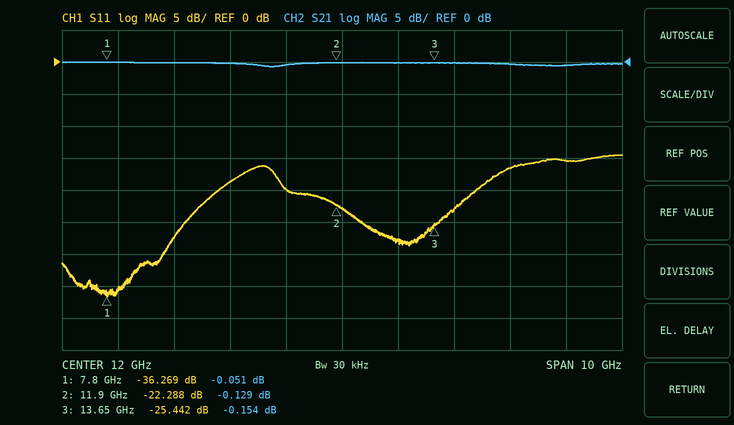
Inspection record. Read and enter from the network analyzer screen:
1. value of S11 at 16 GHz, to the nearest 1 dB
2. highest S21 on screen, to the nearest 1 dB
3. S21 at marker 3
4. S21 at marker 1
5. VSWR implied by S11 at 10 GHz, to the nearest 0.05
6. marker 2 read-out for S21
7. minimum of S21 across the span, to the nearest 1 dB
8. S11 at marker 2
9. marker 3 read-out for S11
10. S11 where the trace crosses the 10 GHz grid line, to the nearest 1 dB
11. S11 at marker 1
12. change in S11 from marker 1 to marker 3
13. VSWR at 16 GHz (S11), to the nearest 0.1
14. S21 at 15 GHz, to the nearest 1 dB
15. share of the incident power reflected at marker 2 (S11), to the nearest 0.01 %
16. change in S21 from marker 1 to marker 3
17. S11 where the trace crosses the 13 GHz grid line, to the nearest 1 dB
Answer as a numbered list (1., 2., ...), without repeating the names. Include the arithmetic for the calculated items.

1. -15 dB
2. 0 dB
3. -0.154 dB
4. -0.051 dB
5. |Γ| = 10^(-19/20) = 0.1122; VSWR = (1 + 0.1122)/(1 − 0.1122) ≈ 1.25
6. -0.129 dB
7. -1 dB
8. -22.288 dB
9. -25.442 dB
10. -19 dB
11. -36.269 dB
12. -25.442 − (-36.269) = 10.827 dB
13. |Γ| = 10^(-15/20) = 0.1778; VSWR = (1 + 0.1778)/(1 − 0.1778) ≈ 1.4
14. 0 dB
15. 10^(-22.288/10) ≈ 0.59 %
16. -0.154 − (-0.051) = -0.103 dB
17. -28 dB
